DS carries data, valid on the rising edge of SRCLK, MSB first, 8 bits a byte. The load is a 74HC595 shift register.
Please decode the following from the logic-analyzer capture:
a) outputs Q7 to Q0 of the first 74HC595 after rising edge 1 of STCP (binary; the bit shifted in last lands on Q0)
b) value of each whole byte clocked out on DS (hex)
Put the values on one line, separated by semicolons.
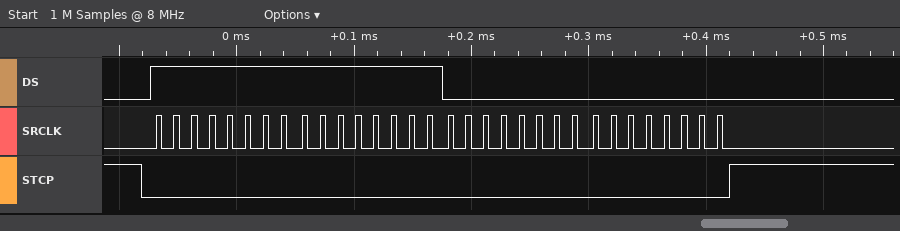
00000000; 0xFF 0xFF 0x00 0x00
